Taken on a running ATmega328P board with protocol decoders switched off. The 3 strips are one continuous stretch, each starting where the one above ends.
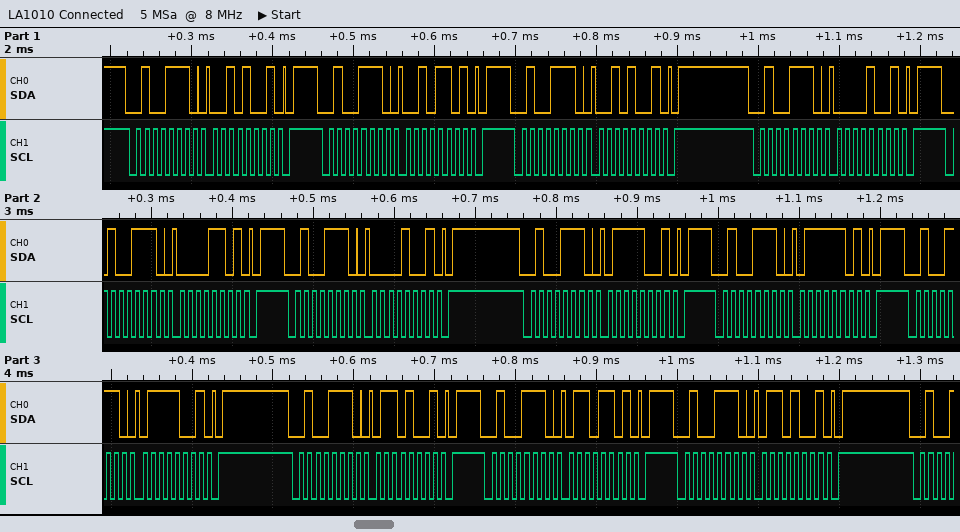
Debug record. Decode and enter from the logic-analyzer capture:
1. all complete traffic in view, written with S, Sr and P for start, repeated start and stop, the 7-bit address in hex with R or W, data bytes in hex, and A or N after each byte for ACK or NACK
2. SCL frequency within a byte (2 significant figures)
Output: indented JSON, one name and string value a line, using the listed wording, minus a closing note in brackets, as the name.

{
  "all complete traffic in view, written with S, Sr and P for start, repeated start and stop, the 7-bit address in hex with R or W, data bytes in hex, and A or N after each byte for ACK or NACK": "S 27W A 29 A P S 27W A 2D A P S 27W A 29 A P S 27W A 09 A P S 27W A 0D A P S 27W A 09 A P S 27W A 79 A P S 27W A 7D A P S 27W A 79 A P S 27W A 69 A P S 27W A 6D A P S 27W A 69 A P",
  "SCL frequency within a byte": "100 kHz"
}
